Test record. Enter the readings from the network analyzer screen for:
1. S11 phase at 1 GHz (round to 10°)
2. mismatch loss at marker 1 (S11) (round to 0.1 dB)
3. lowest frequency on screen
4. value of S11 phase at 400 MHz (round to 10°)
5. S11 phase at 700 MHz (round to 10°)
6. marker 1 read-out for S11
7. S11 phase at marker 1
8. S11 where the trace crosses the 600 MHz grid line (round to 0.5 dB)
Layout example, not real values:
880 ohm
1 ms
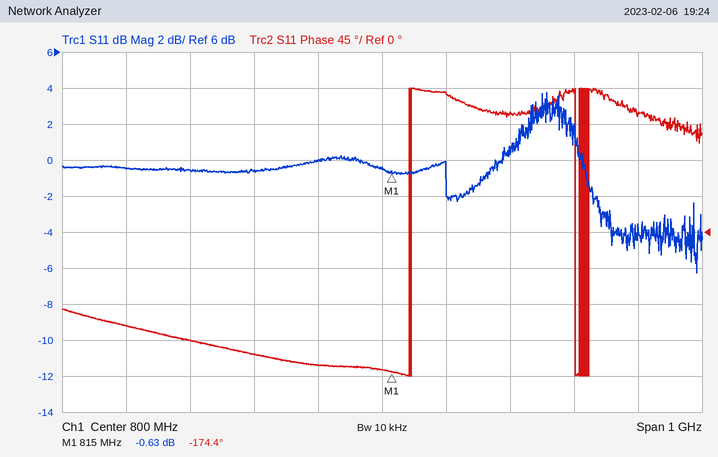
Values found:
150°
8.7 dB
300 MHz
-120°
-170°
-0.63 dB
-174.4°
-0.5 dB
